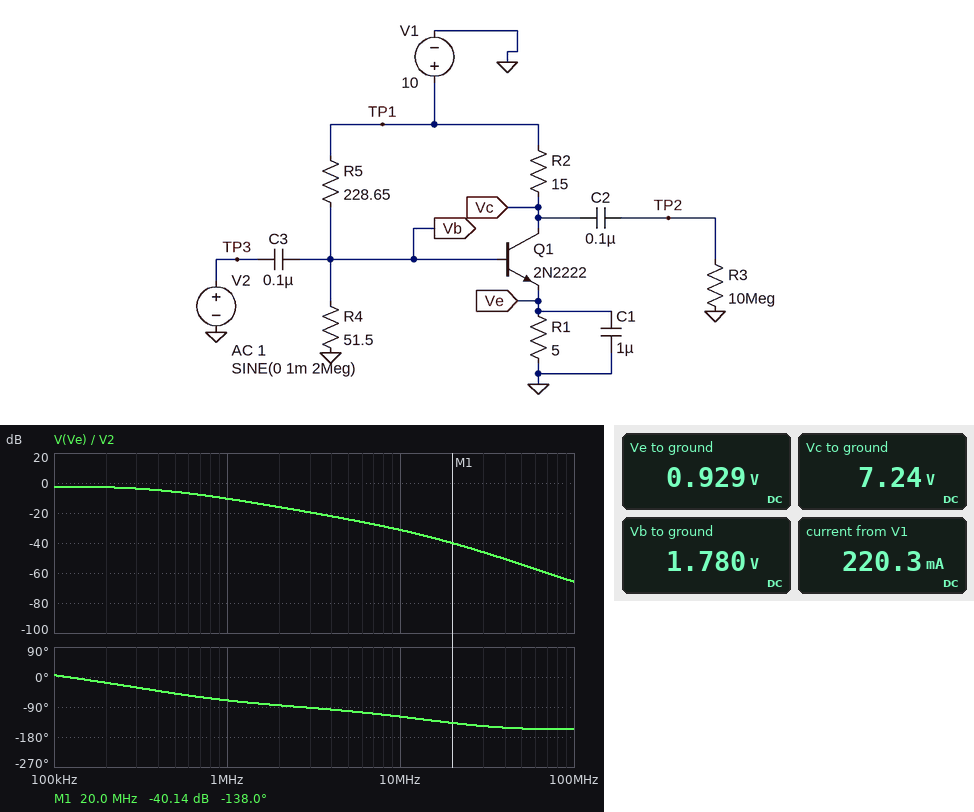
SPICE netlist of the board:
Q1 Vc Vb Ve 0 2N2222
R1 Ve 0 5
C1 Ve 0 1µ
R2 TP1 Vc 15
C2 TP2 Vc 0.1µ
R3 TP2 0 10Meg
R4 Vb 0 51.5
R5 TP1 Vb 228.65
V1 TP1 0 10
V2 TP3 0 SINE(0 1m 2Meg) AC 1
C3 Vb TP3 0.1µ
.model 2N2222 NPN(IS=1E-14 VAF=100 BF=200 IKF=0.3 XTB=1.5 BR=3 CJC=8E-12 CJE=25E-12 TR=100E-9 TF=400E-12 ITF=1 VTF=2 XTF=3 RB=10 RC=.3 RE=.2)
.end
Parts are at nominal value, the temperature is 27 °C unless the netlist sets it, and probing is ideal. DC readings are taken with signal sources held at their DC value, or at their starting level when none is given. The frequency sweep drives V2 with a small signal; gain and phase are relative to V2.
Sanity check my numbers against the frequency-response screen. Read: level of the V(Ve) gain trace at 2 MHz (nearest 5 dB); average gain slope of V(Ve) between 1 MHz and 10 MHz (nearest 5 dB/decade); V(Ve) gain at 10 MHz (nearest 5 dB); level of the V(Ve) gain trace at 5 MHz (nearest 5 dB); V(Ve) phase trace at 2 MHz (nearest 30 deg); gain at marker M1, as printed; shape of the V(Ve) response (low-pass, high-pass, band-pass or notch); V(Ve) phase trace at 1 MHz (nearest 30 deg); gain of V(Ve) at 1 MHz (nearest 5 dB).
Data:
-15 dB
-20 dB/decade
-30 dB
-25 dB
-90 deg
-40.14 dB
low-pass
-60 deg
-10 dB
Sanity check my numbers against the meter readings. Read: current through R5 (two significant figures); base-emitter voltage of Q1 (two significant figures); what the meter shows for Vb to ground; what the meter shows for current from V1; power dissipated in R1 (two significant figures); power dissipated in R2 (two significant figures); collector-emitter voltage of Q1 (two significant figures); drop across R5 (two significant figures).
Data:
36 mA
850 mV
1.780 V
220.3 mA
170 mW
510 mW
6.3 V
8.2 V
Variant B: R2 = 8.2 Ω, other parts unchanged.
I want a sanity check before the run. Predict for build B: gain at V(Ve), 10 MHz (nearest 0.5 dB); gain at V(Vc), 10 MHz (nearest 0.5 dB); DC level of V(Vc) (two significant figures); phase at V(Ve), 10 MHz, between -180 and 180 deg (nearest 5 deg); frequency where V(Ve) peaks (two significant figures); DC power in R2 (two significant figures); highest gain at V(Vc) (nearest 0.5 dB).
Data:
-31.0 dB
23.0 dB
8.5 V
-115 deg
120 kHz
280 mW
24.0 dB
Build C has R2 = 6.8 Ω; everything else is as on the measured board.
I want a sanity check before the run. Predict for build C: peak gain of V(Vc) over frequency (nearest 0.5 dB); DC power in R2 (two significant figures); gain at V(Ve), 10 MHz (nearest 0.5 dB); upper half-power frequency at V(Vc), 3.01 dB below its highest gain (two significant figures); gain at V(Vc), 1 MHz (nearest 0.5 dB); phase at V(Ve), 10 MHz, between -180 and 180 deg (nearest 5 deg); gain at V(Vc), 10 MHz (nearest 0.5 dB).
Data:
22.5 dB
230 mW
-31.0 dB
18 MHz
22.0 dB
-115 deg
21.5 dB
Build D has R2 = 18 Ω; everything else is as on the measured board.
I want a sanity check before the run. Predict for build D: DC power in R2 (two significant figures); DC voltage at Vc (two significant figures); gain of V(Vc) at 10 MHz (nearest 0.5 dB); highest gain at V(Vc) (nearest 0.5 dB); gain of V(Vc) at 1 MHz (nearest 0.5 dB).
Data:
610 mW
6.7 V
29.5 dB
31.0 dB
30.5 dB
